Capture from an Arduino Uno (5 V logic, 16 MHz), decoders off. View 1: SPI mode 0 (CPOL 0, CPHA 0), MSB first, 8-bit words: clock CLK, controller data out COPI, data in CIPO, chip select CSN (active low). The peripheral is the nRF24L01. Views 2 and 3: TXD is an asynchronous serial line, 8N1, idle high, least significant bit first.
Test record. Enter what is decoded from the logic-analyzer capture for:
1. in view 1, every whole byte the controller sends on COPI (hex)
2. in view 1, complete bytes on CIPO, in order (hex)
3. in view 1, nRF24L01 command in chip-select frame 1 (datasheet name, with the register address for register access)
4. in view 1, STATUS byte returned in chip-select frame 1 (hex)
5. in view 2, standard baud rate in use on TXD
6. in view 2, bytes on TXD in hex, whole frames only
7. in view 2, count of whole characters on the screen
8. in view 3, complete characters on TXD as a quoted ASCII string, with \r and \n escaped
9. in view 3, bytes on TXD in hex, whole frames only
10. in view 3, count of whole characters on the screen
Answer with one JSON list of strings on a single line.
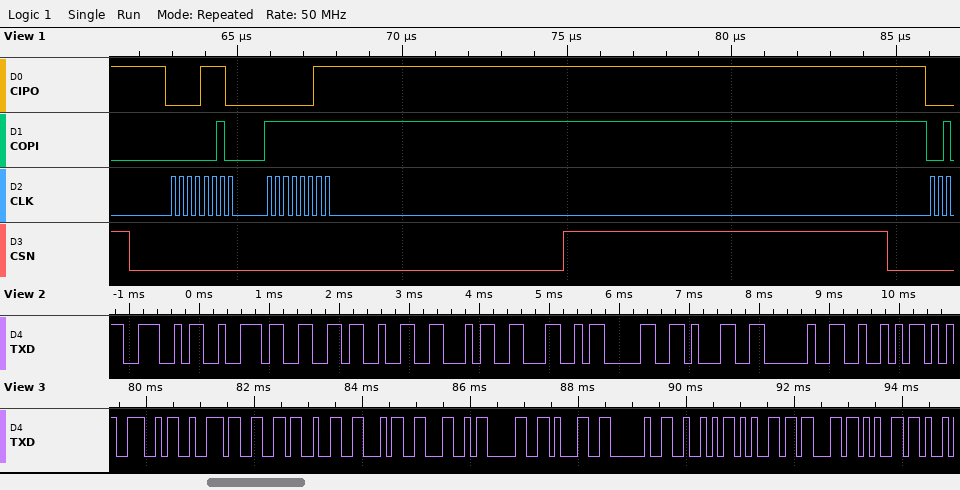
["02 FF", "0E 03", "R_REGISTER 0x02", "0x0E", "9600 baud", "4E 72 66 32 34 4C 30 31 20 52", "10", "\"Nrf24L01 Rece\"", "4E 72 66 32 34 4C 30 31 20 52 65 63 65", "13"]
